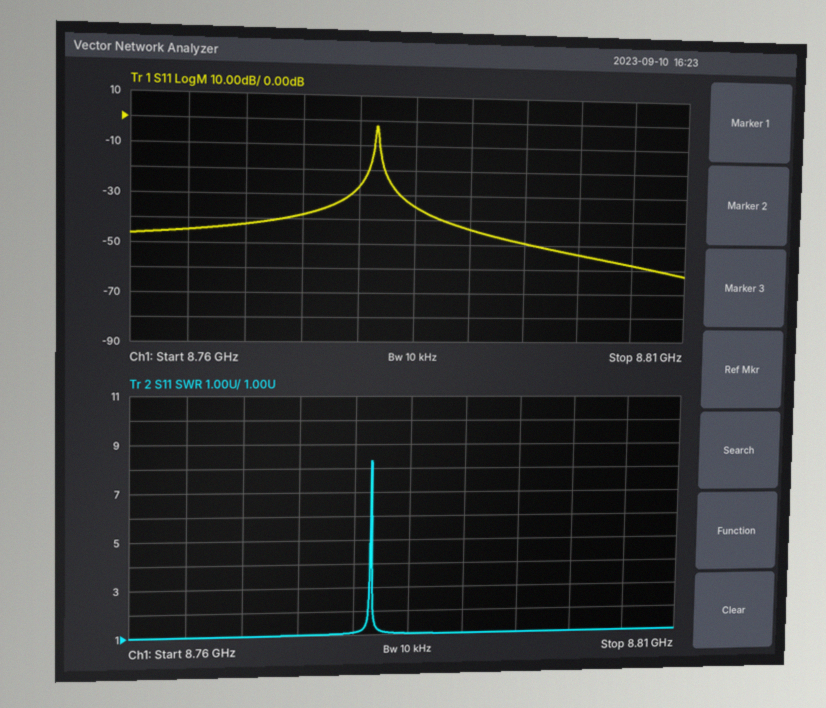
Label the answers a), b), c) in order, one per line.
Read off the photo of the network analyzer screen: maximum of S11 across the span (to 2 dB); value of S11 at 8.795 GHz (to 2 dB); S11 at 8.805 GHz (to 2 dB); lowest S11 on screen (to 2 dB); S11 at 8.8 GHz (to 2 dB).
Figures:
a) -2 dB
b) -50 dB
c) -58 dB
d) -62 dB
e) -54 dB
